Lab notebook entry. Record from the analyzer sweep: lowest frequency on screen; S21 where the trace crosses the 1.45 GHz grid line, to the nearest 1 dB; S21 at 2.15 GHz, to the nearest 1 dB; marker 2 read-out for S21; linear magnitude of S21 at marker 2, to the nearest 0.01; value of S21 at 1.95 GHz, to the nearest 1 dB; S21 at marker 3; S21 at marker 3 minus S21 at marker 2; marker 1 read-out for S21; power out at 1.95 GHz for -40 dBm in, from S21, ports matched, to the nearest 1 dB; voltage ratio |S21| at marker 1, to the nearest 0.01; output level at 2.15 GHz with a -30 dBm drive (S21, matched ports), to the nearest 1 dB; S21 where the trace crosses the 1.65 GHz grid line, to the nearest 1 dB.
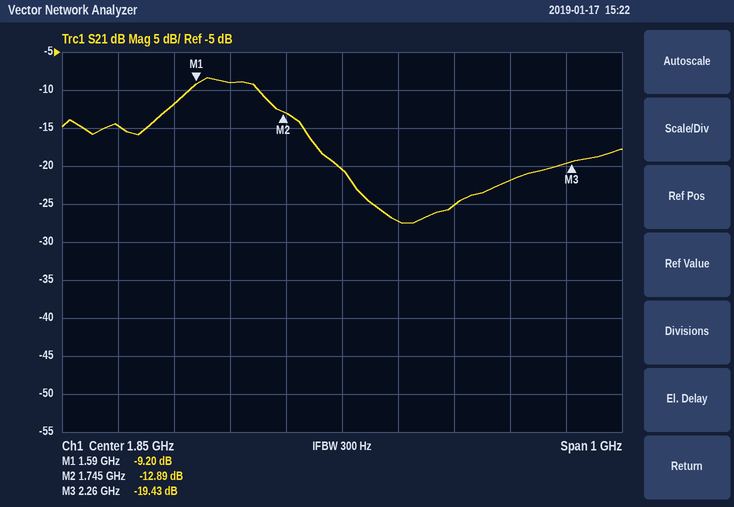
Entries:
1.35 GHz
-15 dB
-22 dB
-12.89 dB
0.23
-27 dB
-19.43 dB
-6.54 dB
-9.20 dB
-67 dBm
0.35
-52 dBm
-9 dB
